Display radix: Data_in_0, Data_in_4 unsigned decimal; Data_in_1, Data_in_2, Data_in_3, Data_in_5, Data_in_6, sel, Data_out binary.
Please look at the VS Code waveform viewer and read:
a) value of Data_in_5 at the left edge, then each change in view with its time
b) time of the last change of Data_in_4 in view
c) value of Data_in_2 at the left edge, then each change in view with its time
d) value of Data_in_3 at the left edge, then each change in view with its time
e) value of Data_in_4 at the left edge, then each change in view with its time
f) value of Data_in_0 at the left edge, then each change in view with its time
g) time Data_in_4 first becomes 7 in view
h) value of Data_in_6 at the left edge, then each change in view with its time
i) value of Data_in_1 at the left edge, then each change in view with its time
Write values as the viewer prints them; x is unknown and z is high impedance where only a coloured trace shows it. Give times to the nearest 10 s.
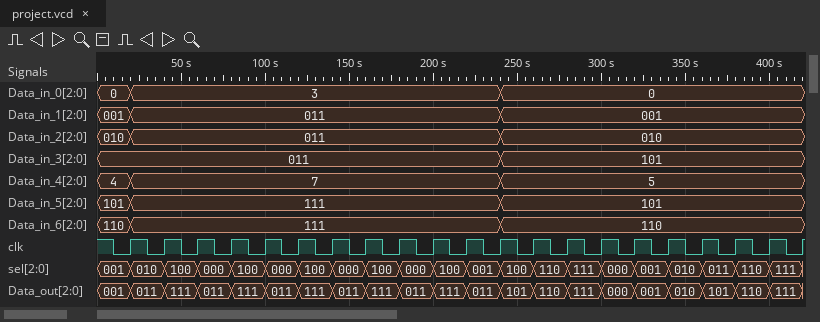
101, 111 at 20 s, 101 at 240 s
240 s
010, 011 at 20 s, 010 at 240 s
011, 101 at 240 s
4, 7 at 20 s, 5 at 240 s
0, 3 at 20 s, 0 at 240 s
20 s
110, 111 at 20 s, 110 at 240 s
001, 011 at 20 s, 001 at 240 s
